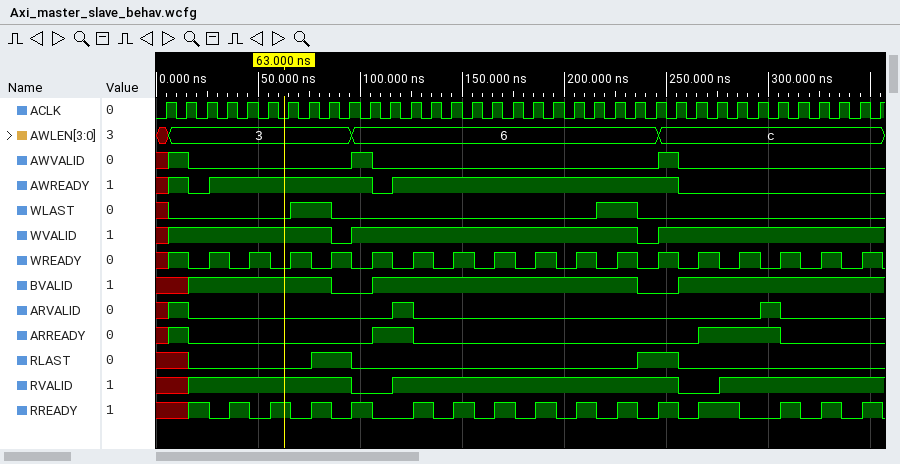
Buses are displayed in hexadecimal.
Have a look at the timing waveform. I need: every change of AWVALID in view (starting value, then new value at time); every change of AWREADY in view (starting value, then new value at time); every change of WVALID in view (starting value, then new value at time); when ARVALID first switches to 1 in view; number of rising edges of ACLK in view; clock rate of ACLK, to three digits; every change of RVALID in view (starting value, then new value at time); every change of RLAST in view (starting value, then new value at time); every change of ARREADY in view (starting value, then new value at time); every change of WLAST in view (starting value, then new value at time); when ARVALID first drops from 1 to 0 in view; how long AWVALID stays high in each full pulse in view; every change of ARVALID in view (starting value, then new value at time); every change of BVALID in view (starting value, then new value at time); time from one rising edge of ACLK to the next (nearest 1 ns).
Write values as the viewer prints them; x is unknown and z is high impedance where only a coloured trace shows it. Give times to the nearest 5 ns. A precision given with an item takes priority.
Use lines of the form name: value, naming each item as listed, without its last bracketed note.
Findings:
every change of AWVALID in view: x, 1 at 5 ns, 0 at 15 ns, 1 at 95 ns, 0 at 105 ns, 1 at 245 ns, 0 at 255 ns
every change of AWREADY in view: x, 1 at 5 ns, 0 at 15 ns, 1 at 25 ns, 0 at 105 ns, 1 at 115 ns, 0 at 255 ns
every change of WVALID in view: x, 1 at 5 ns, 0 at 85 ns, 1 at 95 ns, 0 at 235 ns, 1 at 245 ns
when ARVALID first switches to 1 in view: 5 ns
number of rising edges of ACLK in view: 36
clock rate of ACLK, to three digits: 100 MHz
every change of RVALID in view: x, 1 at 15 ns, 0 at 95 ns, 1 at 115 ns, 0 at 255 ns, 1 at 275 ns
every change of RLAST in view: x, 0 at 15 ns, 1 at 75 ns, 0 at 95 ns, 1 at 235 ns, 0 at 255 ns
every change of ARREADY in view: x, 1 at 5 ns, 0 at 15 ns, 1 at 105 ns, 0 at 125 ns, 1 at 265 ns, 0 at 305 ns
every change of WLAST in view: x, 0 at 5 ns, 1 at 65 ns, 0 at 85 ns, 1 at 215 ns, 0 at 235 ns
when ARVALID first drops from 1 to 0 in view: 15 ns
how long AWVALID stays high in each full pulse in view: 10 ns, 10 ns
every change of ARVALID in view: x, 1 at 5 ns, 0 at 15 ns, 1 at 115 ns, 0 at 125 ns, 1 at 295 ns, 0 at 305 ns
every change of BVALID in view: x, 1 at 15 ns, 0 at 85 ns, 1 at 105 ns, 0 at 235 ns, 1 at 255 ns
time from one rising edge of ACLK to the next: 10 ns
